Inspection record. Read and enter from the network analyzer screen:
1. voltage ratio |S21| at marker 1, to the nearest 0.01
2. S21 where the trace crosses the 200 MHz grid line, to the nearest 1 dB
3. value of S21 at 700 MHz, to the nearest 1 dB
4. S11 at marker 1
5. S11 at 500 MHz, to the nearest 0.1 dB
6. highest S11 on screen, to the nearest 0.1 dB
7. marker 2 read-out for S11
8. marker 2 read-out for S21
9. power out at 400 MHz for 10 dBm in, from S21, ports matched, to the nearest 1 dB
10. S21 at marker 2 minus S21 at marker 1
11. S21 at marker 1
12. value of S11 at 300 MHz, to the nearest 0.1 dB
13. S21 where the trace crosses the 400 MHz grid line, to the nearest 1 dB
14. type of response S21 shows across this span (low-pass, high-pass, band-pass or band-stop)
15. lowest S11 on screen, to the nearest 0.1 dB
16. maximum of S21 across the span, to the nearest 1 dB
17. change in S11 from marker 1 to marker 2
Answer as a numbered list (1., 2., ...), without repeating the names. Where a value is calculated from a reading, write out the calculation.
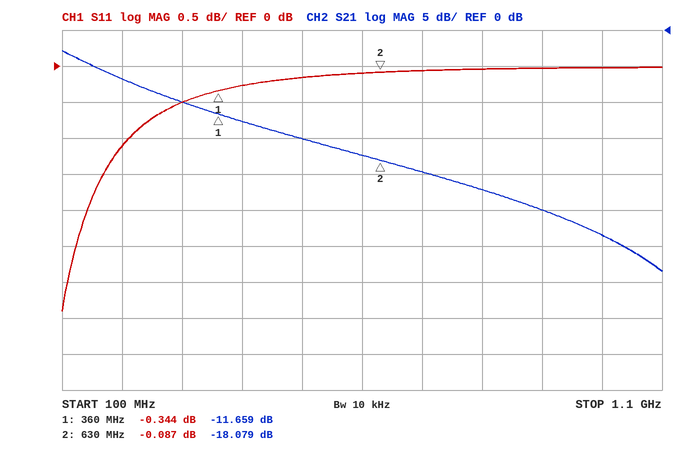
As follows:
1. 10^(-11.659/20) ≈ 0.26
2. -7 dB
3. -20 dB
4. -0.344 dB
5. -0.2 dB
6. 0.0 dB
7. -0.087 dB
8. -18.079 dB
9. 10 dBm + (-13 dB) = -3 dBm
10. -18.079 − (-11.659) = -6.420 dB
11. -11.659 dB
12. -0.5 dB
13. -13 dB
14. low-pass
15. -3.4 dB
16. -3 dB
17. -0.087 − (-0.344) = 0.257 dB
